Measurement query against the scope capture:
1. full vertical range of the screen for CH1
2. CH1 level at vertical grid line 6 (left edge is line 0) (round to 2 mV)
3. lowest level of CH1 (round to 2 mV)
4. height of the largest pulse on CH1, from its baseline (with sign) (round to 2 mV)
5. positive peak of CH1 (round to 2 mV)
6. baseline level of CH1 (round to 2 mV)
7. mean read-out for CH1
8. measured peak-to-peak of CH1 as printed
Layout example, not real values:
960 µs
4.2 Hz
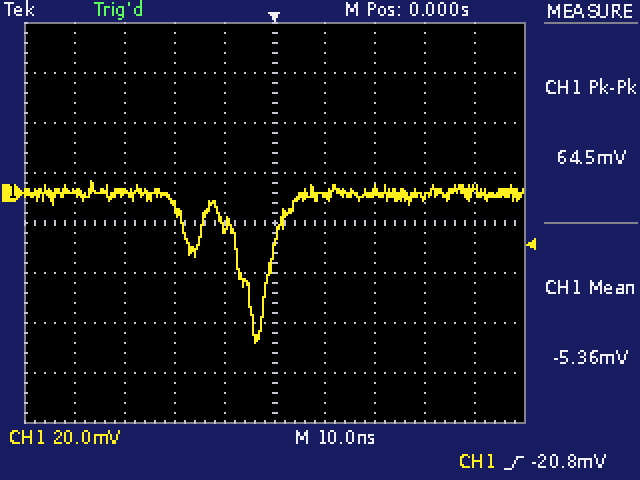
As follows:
160 mV
-2 mV
-60 mV
-60 mV
4 mV
0 mV
-5.36 mV
64.5 mV
